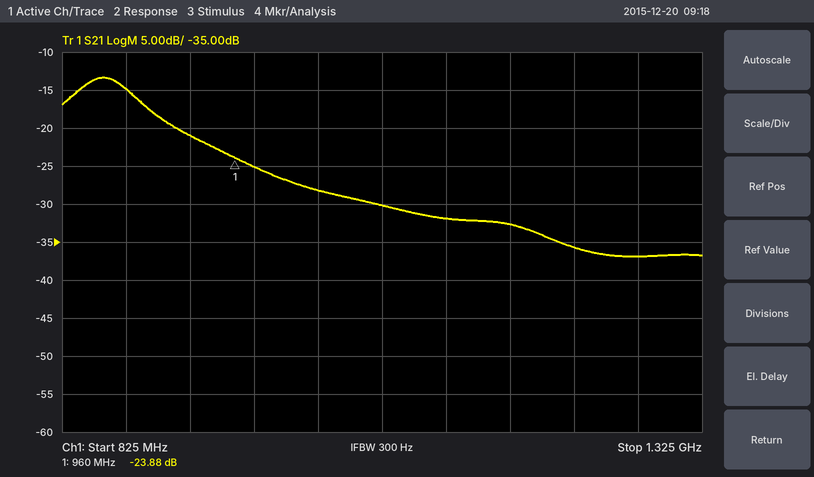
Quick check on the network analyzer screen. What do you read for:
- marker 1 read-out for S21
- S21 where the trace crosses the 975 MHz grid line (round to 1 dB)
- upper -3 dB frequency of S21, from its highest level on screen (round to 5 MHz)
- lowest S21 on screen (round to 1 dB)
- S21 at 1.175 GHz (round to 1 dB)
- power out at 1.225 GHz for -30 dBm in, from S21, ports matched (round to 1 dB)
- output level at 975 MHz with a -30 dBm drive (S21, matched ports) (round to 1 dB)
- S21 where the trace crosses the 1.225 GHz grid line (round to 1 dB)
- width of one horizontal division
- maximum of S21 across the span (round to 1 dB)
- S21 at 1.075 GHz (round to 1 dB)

-23.88 dB
-25 dB
885 MHz
-37 dB
-33 dB
-66 dBm
-55 dBm
-36 dB
50 MHz
-13 dB
-30 dB
